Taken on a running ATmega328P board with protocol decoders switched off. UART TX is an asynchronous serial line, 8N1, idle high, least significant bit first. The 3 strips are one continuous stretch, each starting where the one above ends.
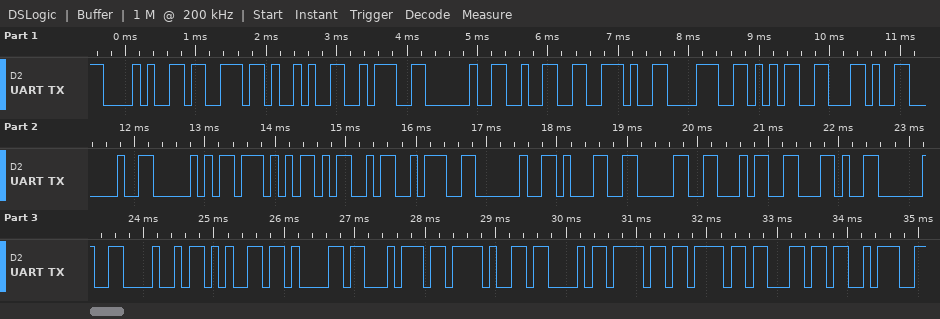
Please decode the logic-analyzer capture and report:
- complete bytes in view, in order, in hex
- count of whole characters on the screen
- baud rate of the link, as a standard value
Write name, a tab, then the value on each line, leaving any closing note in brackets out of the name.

complete bytes in view, in order, in hex	28 73 29 3A 20 32 2E 38 35 2C 20 50 57 4D 3A 20 31 30 34 2C 20 48 65 61 74 2F 43 6F 6F 6C 3A
count of whole characters on the screen	31
baud rate of the link, as a standard value	9600 baud
